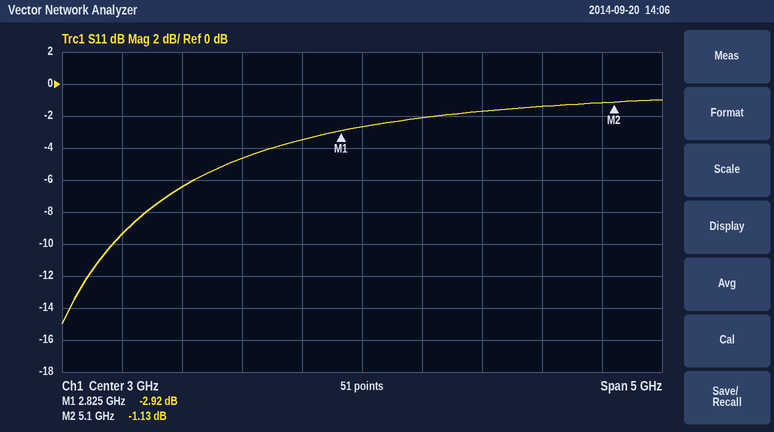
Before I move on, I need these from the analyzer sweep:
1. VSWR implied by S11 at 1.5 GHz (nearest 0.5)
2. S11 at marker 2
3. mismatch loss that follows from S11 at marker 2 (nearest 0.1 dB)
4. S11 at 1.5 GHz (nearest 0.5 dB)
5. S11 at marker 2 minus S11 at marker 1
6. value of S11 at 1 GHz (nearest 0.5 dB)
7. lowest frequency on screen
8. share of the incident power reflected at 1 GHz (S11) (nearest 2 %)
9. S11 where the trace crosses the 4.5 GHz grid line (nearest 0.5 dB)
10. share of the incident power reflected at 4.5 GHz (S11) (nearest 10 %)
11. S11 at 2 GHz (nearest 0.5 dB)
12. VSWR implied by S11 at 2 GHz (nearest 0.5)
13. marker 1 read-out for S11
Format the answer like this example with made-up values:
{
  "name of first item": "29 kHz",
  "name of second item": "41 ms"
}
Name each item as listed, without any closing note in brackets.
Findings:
{
  "VSWR implied by S11 at 1.5 GHz": "3.0",
  "S11 at marker 2": "-1.13 dB",
  "mismatch loss that follows from S11 at marker 2": "6.4 dB",
  "S11 at 1.5 GHz": "-6.5 dB",
  "S11 at marker 2 minus S11 at marker 1": "1.79 dB",
  "value of S11 at 1 GHz": "-9.5 dB",
  "lowest frequency on screen": "500 MHz",
  "share of the incident power reflected at 1 GHz (S11)": "12 %",
  "S11 where the trace crosses the 4.5 GHz grid line": "-1.5 dB",
  "share of the incident power reflected at 4.5 GHz (S11)": "70 %",
  "S11 at 2 GHz": "-4.5 dB",
  "VSWR implied by S11 at 2 GHz": "4.0",
  "marker 1 read-out for S11": "-2.92 dB"
}
